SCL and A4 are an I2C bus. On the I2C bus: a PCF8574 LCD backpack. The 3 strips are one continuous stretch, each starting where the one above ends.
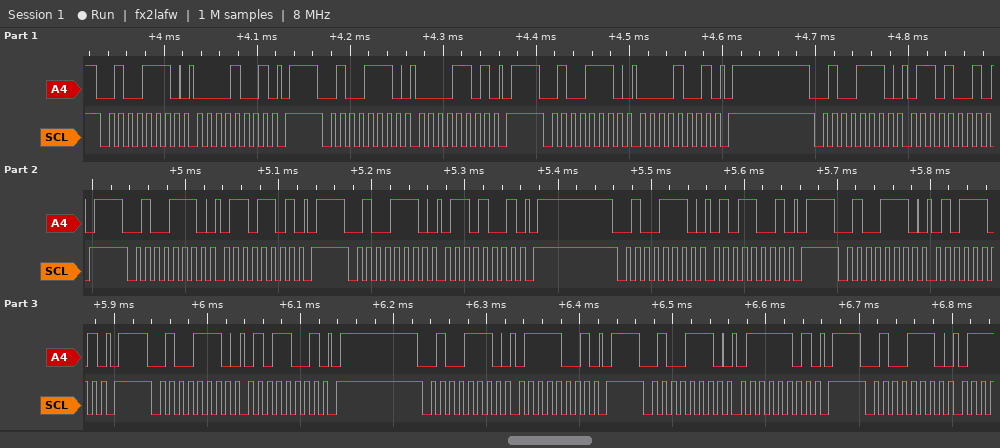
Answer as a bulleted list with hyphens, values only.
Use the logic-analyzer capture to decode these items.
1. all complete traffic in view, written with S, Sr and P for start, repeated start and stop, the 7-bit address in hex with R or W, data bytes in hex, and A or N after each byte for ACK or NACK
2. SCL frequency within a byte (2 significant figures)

- S 27W A 09 A P S 27W A 0D A P S 27W A 09 A P S 27W A 69 A P S 27W A 6D A P S 27W A 69 A P S 27W A 59 A P S 27W A 5D A P S 27W A 59 A P S 27W A 79 A P S 27W A 7D A P S 27W A
- 100 kHz
